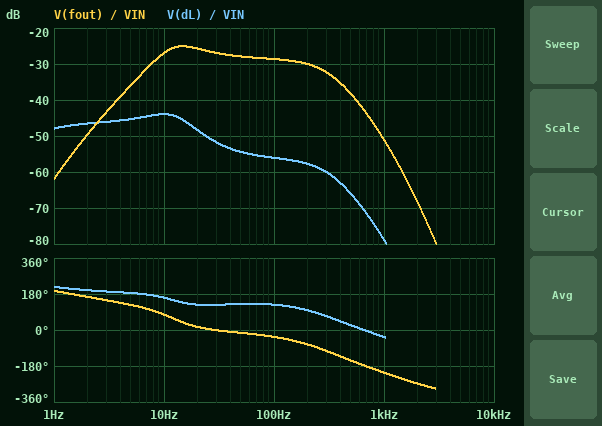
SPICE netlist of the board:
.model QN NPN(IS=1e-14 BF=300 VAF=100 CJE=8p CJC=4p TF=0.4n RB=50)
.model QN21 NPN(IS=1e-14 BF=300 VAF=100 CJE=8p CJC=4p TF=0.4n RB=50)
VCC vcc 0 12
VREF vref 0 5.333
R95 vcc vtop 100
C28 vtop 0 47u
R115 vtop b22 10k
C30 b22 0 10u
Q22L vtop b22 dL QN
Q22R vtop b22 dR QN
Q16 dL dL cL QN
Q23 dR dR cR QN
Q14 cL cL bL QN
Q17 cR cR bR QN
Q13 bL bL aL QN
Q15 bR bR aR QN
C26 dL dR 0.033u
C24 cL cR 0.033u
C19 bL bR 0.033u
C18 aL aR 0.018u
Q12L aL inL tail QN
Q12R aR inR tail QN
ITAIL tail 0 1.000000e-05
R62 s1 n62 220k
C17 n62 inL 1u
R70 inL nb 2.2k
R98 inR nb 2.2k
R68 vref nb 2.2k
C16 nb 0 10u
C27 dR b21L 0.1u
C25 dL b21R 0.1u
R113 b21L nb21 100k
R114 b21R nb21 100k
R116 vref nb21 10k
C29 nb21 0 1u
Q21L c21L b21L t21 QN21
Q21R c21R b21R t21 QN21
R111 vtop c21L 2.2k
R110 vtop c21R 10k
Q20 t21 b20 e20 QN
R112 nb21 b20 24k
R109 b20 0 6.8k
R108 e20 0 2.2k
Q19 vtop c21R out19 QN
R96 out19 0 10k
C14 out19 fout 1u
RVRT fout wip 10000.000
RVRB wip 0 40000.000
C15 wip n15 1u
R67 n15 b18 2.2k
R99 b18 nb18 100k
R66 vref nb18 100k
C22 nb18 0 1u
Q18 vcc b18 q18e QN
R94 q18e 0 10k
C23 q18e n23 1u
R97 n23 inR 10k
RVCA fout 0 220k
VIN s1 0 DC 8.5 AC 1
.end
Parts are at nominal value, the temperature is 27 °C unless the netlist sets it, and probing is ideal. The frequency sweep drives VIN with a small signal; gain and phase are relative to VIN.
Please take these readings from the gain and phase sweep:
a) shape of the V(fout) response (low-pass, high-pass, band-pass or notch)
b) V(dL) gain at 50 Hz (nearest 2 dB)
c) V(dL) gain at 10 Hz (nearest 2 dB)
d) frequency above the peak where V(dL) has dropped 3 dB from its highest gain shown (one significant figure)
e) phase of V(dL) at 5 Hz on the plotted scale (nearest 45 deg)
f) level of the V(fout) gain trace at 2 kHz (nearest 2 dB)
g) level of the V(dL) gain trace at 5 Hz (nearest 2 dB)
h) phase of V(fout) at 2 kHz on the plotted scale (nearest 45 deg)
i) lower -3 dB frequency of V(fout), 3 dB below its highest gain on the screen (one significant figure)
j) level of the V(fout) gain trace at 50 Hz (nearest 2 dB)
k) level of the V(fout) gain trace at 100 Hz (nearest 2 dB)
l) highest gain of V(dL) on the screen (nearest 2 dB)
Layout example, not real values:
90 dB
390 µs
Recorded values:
band-pass
-54 dB
-44 dB
20 Hz
180 deg
-68 dB
-46 dB
-270 deg
9 Hz
-28 dB
-28 dB
-44 dB
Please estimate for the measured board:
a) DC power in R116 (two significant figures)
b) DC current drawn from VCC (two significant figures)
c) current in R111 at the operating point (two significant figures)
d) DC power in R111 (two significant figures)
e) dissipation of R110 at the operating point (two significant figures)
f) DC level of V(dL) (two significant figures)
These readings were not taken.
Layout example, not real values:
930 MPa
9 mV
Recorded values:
170 µW
1.6 mA
64 µA
9.1 µW
46 µW
11 V
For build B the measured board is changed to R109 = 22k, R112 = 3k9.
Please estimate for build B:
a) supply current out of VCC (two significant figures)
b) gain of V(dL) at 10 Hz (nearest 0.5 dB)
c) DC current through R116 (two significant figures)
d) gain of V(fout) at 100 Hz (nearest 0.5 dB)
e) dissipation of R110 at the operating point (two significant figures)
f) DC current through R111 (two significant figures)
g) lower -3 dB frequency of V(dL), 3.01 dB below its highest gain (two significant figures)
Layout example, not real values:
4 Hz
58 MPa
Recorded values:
2.2 mA
-40.5 dB
150 µA
-24.0 dB
3.2 mW
590 µA
6.7 Hz
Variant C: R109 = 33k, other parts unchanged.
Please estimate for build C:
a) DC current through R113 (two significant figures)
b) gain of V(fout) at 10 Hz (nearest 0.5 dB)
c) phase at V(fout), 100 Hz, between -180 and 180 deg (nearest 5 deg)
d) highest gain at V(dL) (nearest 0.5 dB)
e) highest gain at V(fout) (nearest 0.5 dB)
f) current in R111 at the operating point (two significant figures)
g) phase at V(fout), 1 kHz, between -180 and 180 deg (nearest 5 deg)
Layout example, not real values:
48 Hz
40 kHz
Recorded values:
1.4 µA
-18.0 dB
-15 deg
-40.5 dB
-16.5 dB
440 µA
150 deg
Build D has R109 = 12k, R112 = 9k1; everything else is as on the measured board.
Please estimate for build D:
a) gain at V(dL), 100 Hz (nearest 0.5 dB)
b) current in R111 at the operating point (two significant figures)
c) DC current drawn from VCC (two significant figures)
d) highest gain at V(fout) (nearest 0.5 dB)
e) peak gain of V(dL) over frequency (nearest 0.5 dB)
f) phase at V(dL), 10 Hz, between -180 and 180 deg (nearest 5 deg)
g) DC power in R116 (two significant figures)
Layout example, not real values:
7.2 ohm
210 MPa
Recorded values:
-64.0 dB
320 µA
1.9 mA
-17.5 dB
-41.0 dB
155 deg
300 µW
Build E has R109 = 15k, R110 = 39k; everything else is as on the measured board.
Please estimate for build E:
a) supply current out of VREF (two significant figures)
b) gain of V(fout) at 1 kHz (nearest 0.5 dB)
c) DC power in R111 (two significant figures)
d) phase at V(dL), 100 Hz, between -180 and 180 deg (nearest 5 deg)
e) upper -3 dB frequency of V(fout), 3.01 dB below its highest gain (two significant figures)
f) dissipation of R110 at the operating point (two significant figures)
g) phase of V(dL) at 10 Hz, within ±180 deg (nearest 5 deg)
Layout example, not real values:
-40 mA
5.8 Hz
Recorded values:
110 µA
-30.5 dB
120 µW
80 deg
810 Hz
1.7 mW
165 deg
